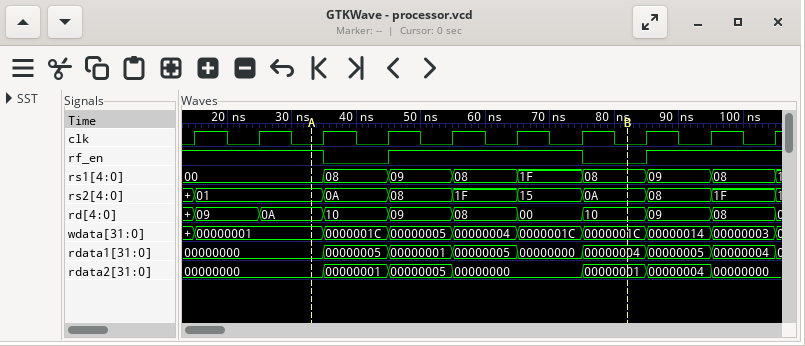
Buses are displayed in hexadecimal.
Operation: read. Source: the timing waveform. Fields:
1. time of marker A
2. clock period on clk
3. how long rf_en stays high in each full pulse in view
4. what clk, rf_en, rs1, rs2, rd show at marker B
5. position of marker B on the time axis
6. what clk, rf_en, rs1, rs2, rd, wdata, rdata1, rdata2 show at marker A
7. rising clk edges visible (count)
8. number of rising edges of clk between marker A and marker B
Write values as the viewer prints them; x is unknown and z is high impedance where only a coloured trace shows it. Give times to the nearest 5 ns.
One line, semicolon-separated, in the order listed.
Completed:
35 ns; 10 ns; 30 ns; clk=0, rf_en=0, rs1=08, rs2=0A, rd=10; 80 ns; clk=0, rf_en=1, rs1=00, rs2=01, rd=0A, wdata=00000001, rdata1=00000000, rdata2=00000000; 10; 5
